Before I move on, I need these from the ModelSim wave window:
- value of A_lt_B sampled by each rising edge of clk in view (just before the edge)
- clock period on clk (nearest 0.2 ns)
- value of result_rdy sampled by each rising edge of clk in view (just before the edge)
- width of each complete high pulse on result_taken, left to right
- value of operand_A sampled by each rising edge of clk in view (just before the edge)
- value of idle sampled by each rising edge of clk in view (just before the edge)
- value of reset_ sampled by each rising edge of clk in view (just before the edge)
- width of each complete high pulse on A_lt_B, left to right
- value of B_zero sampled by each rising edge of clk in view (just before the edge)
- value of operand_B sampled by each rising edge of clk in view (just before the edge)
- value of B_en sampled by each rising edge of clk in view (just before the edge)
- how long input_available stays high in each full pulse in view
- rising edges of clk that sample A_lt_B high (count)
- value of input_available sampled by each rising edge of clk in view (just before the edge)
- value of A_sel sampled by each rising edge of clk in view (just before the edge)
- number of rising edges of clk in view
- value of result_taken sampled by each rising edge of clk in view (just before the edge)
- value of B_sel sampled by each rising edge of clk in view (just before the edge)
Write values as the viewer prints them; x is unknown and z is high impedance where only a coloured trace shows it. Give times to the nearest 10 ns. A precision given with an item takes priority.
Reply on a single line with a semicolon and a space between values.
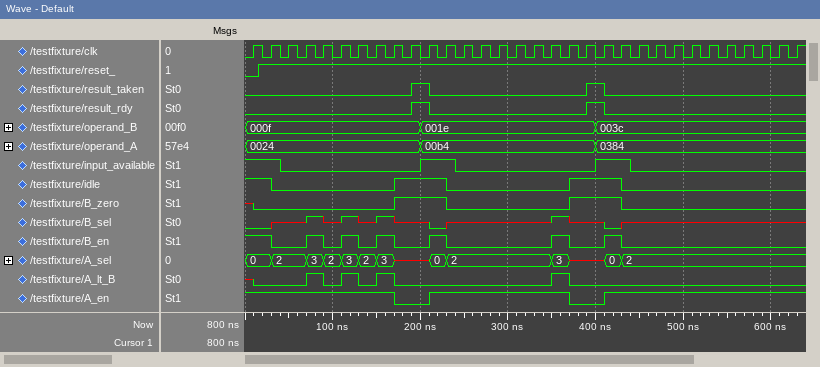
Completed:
x 0 0 0 1 0 1 0 1 0 0 0 0 0 0 0 0 0 1 0 0 0 0 0 0 0 0 0 0 0 0 0; 20 ns; 0 0 0 0 0 0 0 0 0 0 1 0 0 0 0 0 0 0 0 0 1 0 0 0 0 0 0 0 0 0 0 0; 20 ns, 20 ns; 0024, 0024, 0024, 0024, 0024, 0024, 0024, 0024, 0024, 0024, 00b4, 00b4, 00b4, 00b4, 00b4, 00b4, 00b4, 00b4, 00b4, 00b4, 0384, 0384, 0384, 0384, 0384, 0384, 0384, 0384, 0384, 0384, 0384, 0384; 1 1 0 0 0 0 0 0 0 1 1 1 0 0 0 0 0 0 0 1 1 1 0 0 0 0 0 0 0 0 0 0; 0 1 1 1 1 1 1 1 1 1 1 1 1 1 1 1 1 1 1 1 1 1 1 1 1 1 1 1 1 1 1 1; 20 ns, 20 ns, 20 ns, 20 ns; x 0 0 0 0 0 0 0 0 1 1 1 0 0 0 0 0 0 0 1 1 1 0 0 0 0 0 0 0 0 0 0; 000f, 000f, 000f, 000f, 000f, 000f, 000f, 000f, 000f, 000f, 001e, 001e, 001e, 001e, 001e, 001e, 001e, 001e, 001e, 001e, 003c, 003c, 003c, 003c, 003c, 003c, 003c, 003c, 003c, 003c, 003c, 003c; 1 1 0 0 1 0 1 0 1 0 0 1 0 0 0 0 0 0 1 0 0 1 0 0 0 0 0 0 0 0 0 0; 40 ns, 40 ns; 4; 1 1 0 0 0 0 0 0 0 0 1 1 0 0 0 0 0 0 0 0 1 1 0 0 0 0 0 0 0 0 0 0; 0, 0, 2, 2, 3, 2, 3, 2, 3, x, x, 0, 2, 2, 2, 2, 2, 2, 3, x, x, 0, 2, 2, 2, 2, 2, 2, 2, 2, 2, 2; 32; 0 0 0 0 0 0 0 0 0 0 1 0 0 0 0 0 0 0 0 0 1 0 0 0 0 0 0 0 0 0 0 0; 0 0 x x 1 x 1 x 1 x x 0 x x x x x x 1 x x 0 x x x x x x x x x x
